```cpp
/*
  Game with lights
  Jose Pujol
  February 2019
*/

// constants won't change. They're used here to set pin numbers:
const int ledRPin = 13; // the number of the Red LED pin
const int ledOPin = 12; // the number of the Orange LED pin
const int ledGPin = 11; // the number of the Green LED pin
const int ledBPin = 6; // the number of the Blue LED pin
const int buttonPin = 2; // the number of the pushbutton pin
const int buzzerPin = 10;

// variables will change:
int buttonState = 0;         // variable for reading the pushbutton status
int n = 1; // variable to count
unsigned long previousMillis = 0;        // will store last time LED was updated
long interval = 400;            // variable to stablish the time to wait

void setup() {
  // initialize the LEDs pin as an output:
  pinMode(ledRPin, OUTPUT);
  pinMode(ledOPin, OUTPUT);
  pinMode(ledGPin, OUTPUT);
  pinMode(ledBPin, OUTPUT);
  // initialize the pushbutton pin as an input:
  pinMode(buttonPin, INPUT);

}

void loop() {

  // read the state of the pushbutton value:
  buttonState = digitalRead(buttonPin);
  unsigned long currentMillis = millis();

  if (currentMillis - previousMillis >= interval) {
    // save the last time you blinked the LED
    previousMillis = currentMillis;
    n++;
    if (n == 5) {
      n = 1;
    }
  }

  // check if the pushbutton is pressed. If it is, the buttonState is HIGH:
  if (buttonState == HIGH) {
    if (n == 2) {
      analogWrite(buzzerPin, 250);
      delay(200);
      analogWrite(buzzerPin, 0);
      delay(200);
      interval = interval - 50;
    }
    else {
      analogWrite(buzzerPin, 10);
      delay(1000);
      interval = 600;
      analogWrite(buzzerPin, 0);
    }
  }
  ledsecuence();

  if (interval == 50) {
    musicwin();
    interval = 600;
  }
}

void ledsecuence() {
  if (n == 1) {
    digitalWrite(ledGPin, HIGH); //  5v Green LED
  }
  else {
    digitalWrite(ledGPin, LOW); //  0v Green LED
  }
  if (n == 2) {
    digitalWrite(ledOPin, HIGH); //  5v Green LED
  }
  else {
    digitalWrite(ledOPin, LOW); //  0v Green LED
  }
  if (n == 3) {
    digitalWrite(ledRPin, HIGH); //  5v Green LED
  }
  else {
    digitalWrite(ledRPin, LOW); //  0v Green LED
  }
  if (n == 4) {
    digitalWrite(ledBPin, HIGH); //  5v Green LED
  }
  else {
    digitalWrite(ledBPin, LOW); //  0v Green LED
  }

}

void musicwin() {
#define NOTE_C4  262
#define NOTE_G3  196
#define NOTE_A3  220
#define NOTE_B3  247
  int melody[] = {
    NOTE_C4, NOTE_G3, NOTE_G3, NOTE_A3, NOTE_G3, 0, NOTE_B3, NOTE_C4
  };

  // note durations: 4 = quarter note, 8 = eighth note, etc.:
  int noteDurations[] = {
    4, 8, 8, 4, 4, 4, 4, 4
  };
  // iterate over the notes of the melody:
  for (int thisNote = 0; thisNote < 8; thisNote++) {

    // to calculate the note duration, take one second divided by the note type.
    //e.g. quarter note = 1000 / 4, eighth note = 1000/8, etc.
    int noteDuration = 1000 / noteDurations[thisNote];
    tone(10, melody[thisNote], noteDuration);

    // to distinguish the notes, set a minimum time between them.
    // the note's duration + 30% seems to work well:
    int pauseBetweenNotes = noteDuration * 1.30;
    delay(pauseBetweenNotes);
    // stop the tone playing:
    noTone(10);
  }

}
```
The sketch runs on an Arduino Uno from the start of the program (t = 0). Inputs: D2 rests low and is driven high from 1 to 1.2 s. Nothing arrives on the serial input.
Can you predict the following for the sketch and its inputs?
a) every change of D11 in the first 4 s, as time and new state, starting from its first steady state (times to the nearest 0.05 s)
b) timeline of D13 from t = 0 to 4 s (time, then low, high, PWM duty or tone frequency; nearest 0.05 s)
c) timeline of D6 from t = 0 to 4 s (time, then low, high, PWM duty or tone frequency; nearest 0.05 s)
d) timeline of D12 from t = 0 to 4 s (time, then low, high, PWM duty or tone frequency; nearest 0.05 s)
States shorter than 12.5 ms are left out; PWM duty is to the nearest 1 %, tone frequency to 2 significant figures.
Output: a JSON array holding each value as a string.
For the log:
["0 s high; 0.4 s low; 2.6 s high; 3.2 s low", "0 s low; 0.8 s high; 2 s low; 3.8 s high", "0 s low; 2 s high; 2.6 s low", "0 s low; 0.4 s high; 0.8 s low; 3.2 s high; 3.8 s low"]
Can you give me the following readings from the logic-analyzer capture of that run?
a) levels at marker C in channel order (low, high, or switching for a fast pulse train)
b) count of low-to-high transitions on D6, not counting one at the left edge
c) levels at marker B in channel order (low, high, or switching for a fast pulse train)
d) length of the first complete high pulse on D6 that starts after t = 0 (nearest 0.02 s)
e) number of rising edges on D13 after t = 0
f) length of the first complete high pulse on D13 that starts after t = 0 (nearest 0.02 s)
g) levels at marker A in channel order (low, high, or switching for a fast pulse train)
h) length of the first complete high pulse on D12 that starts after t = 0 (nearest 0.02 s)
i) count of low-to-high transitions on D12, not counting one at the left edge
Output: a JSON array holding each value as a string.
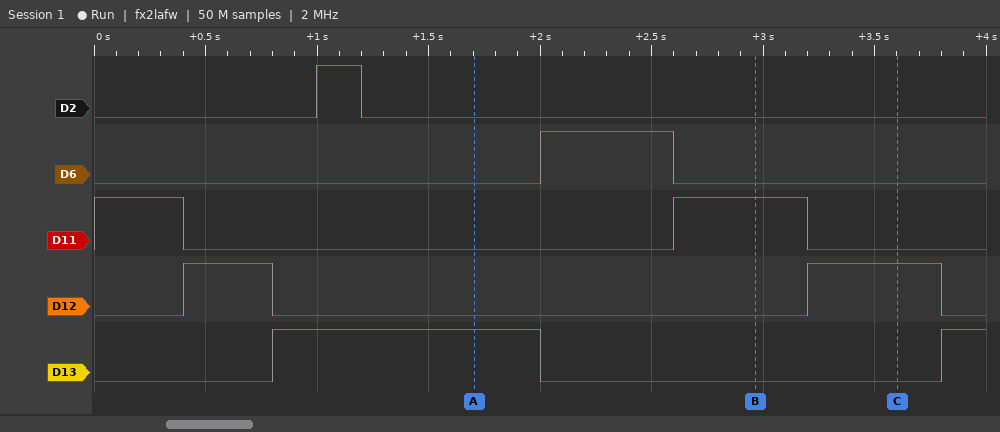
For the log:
["D2 low, D6 low, D11 low, D12 high, D13 low", "1", "D2 low, D6 low, D11 high, D12 low, D13 low", "0.60 s", "2", "1.20 s", "D2 low, D6 low, D11 low, D12 low, D13 high", "0.40 s", "2"]
